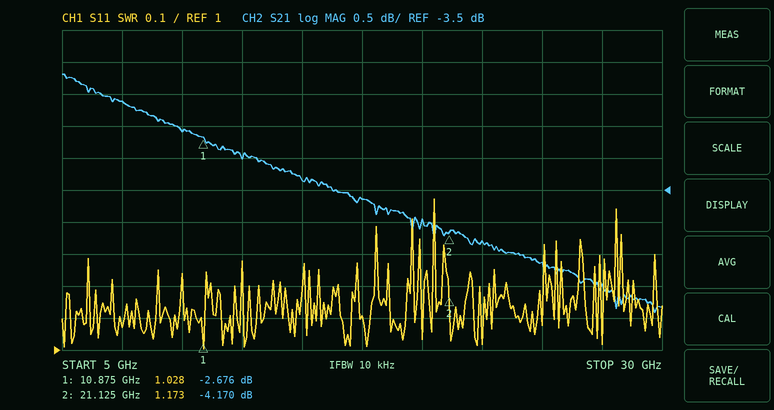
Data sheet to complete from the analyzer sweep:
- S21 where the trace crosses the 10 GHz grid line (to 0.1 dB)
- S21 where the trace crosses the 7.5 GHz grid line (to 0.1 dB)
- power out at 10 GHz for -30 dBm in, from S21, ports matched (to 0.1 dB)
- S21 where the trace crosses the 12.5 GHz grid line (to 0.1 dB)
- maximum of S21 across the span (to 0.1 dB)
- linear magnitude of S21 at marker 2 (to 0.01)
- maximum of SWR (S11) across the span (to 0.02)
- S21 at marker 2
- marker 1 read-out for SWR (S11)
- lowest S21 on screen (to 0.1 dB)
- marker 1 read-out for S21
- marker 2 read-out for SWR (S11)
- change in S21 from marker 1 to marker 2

-2.6 dB
-2.1 dB
-32.6 dBm
-3.0 dB
-1.7 dB
0.62
1.48
-4.170 dB
1.028
-5.4 dB
-2.676 dB
1.173
-1.494 dB
